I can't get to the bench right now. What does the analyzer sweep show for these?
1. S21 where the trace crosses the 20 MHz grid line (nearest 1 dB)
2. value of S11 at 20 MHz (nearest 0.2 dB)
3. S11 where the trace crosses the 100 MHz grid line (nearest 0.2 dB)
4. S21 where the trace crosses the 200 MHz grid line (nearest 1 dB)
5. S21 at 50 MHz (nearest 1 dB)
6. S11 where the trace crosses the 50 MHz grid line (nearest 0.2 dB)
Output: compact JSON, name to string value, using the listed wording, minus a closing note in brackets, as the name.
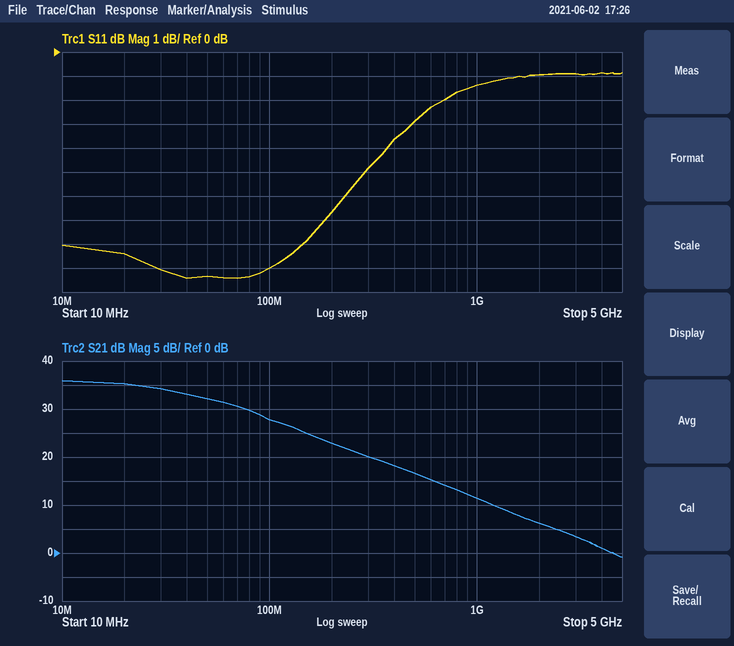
{"S21 where the trace crosses the 20 MHz grid line": "35 dB", "value of S11 at 20 MHz": "-8.4 dB", "S11 where the trace crosses the 100 MHz grid line": "-9.0 dB", "S21 where the trace crosses the 200 MHz grid line": "23 dB", "S21 at 50 MHz": "32 dB", "S11 where the trace crosses the 50 MHz grid line": "-9.4 dB"}
